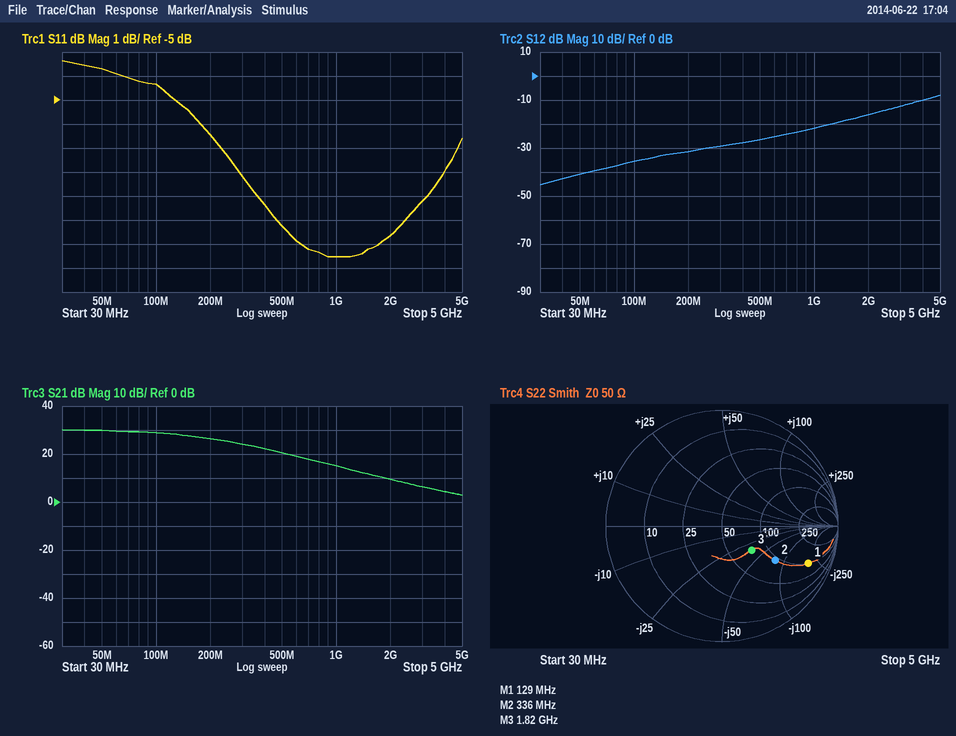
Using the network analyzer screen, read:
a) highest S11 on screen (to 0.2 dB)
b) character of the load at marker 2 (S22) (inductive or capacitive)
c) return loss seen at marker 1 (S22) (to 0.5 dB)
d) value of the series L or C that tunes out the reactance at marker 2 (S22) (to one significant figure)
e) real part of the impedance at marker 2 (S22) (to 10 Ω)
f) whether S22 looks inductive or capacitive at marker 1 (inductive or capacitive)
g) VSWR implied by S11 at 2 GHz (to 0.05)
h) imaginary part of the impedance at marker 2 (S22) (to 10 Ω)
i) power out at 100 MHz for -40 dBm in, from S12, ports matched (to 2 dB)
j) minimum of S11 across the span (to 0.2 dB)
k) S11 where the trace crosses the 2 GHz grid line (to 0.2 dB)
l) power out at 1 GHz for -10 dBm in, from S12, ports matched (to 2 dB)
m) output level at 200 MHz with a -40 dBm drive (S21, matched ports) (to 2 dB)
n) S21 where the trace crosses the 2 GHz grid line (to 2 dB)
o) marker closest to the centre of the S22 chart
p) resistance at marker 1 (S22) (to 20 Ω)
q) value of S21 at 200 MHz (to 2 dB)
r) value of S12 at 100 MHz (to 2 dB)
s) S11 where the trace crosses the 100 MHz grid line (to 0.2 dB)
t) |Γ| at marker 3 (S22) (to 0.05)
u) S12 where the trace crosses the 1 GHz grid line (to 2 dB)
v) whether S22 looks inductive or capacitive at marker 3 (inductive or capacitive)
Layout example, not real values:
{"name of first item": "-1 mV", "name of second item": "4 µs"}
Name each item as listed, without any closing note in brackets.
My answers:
{"highest S11 on screen": "-3.4 dB", "character of the load at marker 2 (S22)": "capacitive", "return loss seen at marker 1 (S22)": "2.0 dB", "value of the series L or C that tunes out the reactance at marker 2 (S22)": "40 nH", "real part of the impedance at marker 2 (S22)": "90 Ω", "whether S22 looks inductive or capacitive at marker 1": "capacitive", "VSWR implied by S11 at 2 GHz": "1.85", "imaginary part of the impedance at marker 2 (S22)": "-80 Ω", "power out at 100 MHz for -40 dBm in, from S12, ports matched": "-76 dBm", "minimum of S11 across the span": "-11.6 dB", "S11 where the trace crosses the 2 GHz grid line": "-10.6 dB", "power out at 1 GHz for -10 dBm in, from S12, ports matched": "-32 dBm", "output level at 200 MHz with a -40 dBm drive (S21, matched ports)": "-14 dBm", "S21 where the trace crosses the 2 GHz grid line": "10 dB", "marker closest to the centre of the S22 chart": "marker 3", "resistance at marker 1 (S22)": "100 Ω", "value of S21 at 200 MHz": "26 dB", "value of S12 at 100 MHz": "-36 dB", "S11 where the trace crosses the 100 MHz grid line": "-4.4 dB", "|Γ| at marker 3 (S22)": "0.35", "S12 where the trace crosses the 1 GHz grid line": "-22 dB", "whether S22 looks inductive or capacitive at marker 3": "capacitive"}
